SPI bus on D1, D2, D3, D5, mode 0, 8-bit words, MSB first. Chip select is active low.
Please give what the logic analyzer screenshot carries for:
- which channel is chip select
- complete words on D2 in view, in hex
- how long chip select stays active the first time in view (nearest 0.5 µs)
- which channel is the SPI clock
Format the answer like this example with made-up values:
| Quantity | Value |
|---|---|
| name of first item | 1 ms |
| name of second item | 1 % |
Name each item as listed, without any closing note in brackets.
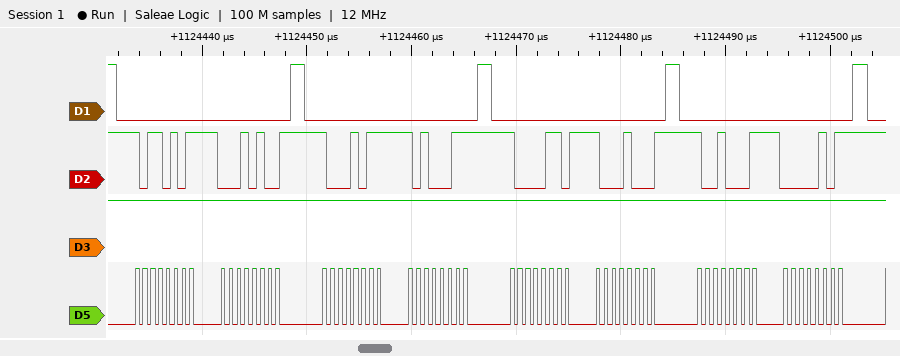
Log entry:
| Quantity | Value |
|---|---|
| which channel is chip select | D1 |
| complete words on D2 in view, in hex | B5, 14, 8B, A3, 86, 88, 91, 05 |
| how long chip select stays active the first time in view | 16.5 µs |
| which channel is the SPI clock | D5 |
